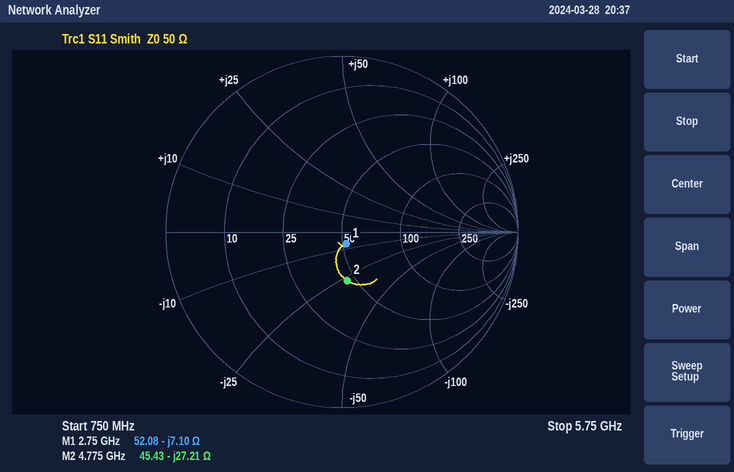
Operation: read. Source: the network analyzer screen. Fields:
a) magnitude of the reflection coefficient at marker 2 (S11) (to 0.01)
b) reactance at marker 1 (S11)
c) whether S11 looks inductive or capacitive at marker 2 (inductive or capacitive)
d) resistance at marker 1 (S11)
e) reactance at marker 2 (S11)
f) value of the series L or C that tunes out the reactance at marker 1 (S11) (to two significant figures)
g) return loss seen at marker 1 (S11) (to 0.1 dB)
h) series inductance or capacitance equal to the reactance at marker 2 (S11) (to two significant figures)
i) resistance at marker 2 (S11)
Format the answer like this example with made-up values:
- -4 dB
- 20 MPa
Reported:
- 0.28
- -7.10 Ω
- capacitive
- 52.08 Ω
- -27.21 Ω
- 410 pH
- 22.8 dB
- 1.2 pF
- 45.43 Ω
